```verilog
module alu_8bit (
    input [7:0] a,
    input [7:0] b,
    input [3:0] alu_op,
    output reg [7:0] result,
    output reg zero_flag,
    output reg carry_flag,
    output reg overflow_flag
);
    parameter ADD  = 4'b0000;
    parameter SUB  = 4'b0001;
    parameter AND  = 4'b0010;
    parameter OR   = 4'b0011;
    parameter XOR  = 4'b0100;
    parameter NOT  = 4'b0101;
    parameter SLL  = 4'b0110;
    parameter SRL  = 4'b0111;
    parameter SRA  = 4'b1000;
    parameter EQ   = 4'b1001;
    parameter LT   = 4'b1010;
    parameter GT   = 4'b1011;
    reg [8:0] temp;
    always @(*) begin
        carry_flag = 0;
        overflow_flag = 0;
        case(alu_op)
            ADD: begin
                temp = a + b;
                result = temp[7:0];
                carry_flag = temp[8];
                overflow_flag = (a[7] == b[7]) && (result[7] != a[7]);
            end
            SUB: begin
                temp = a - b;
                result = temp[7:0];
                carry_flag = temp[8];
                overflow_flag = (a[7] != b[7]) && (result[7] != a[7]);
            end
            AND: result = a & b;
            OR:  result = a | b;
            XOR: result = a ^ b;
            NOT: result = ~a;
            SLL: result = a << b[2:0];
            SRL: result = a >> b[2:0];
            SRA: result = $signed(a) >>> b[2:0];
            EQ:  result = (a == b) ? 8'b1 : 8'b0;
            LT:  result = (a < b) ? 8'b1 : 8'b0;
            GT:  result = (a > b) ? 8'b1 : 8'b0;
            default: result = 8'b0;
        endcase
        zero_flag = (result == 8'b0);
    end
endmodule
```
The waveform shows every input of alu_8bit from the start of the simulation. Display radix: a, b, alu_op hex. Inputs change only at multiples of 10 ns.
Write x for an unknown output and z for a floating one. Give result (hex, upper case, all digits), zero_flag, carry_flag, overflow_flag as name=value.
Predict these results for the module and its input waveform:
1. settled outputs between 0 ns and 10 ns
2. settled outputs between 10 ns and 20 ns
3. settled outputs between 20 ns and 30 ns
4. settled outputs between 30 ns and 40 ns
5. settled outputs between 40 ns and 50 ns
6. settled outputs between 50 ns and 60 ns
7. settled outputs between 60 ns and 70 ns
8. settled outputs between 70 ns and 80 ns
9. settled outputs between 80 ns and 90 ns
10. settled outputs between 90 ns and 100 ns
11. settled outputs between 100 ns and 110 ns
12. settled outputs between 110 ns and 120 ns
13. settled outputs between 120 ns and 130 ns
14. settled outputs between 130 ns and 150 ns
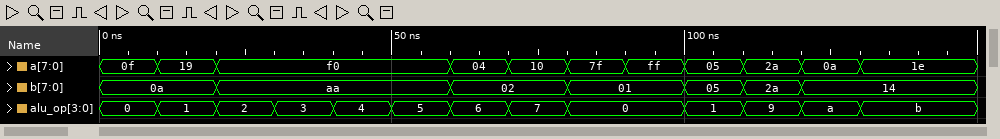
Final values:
result=19, zero_flag=0, carry_flag=0, overflow_flag=0
result=0F, zero_flag=0, carry_flag=0, overflow_flag=0
result=A0, zero_flag=0, carry_flag=0, overflow_flag=0
result=FA, zero_flag=0, carry_flag=0, overflow_flag=0
result=5A, zero_flag=0, carry_flag=0, overflow_flag=0
result=0F, zero_flag=0, carry_flag=0, overflow_flag=0
result=10, zero_flag=0, carry_flag=0, overflow_flag=0
result=04, zero_flag=0, carry_flag=0, overflow_flag=0
result=80, zero_flag=0, carry_flag=0, overflow_flag=1
result=00, zero_flag=1, carry_flag=1, overflow_flag=0
result=00, zero_flag=1, carry_flag=0, overflow_flag=0
result=01, zero_flag=0, carry_flag=0, overflow_flag=0
result=01, zero_flag=0, carry_flag=0, overflow_flag=0
result=01, zero_flag=0, carry_flag=0, overflow_flag=0
